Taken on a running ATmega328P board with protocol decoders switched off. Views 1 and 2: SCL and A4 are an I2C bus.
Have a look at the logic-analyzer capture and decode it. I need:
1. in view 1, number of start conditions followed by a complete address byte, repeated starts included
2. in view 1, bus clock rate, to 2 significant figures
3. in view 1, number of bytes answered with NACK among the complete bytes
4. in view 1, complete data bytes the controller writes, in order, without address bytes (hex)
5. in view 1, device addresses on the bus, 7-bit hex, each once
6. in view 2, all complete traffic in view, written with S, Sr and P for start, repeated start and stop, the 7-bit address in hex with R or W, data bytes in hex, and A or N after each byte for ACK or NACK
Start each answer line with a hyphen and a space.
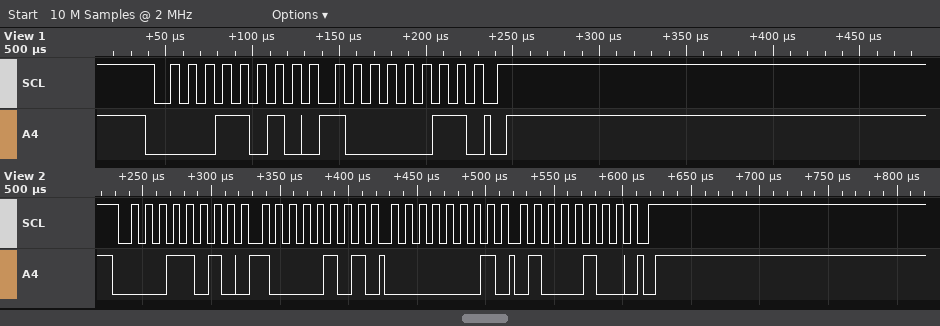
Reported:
- 1
- 100 kHz
- 0
- 83
- 0x0D
- S 0DW A 85 A 01 A 44 A P
